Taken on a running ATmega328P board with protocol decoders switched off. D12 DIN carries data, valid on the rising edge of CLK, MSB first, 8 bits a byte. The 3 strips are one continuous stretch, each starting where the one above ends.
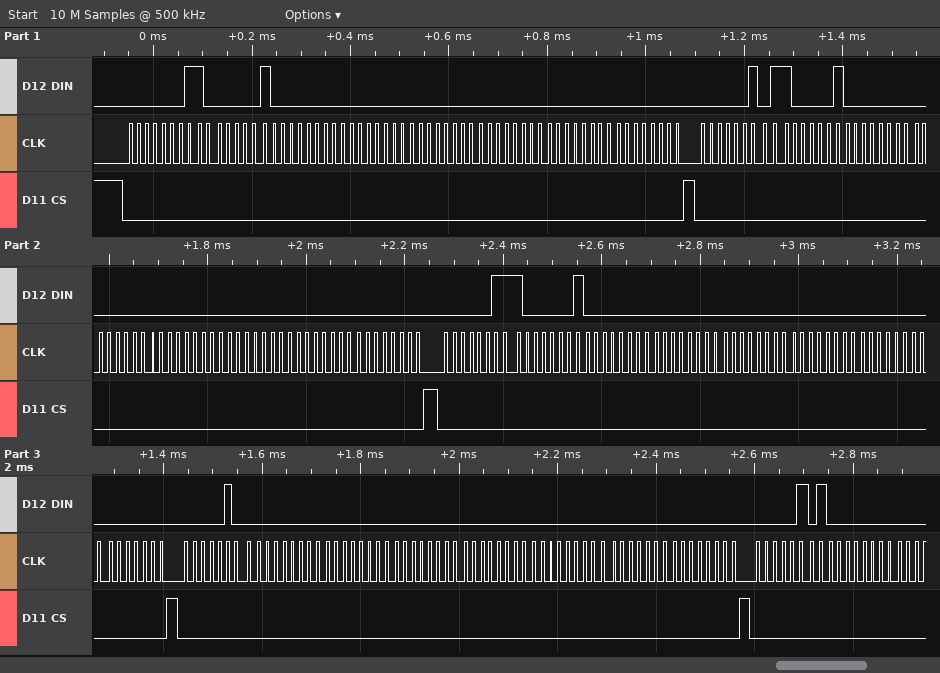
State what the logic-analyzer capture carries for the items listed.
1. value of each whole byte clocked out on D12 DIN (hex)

01 81 00 00 00 00 00 00 02 C1 00 00 00 00 00 00 03 81 00 00 00 00 00 00 04 00 00 00 00 00 00 00 05 00
